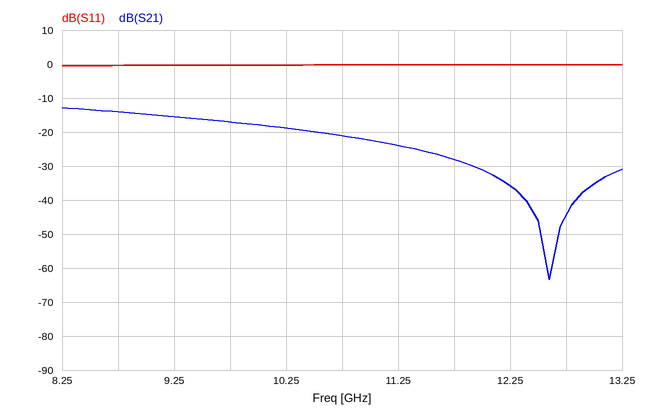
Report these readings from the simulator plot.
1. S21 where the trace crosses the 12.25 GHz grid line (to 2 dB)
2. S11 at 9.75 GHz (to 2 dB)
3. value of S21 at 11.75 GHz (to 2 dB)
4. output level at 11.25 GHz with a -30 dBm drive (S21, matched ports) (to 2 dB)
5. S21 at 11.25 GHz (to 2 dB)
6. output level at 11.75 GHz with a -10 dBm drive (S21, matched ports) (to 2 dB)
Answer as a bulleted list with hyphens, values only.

- -36 dB
- 0 dB
- -28 dB
- -54 dBm
- -24 dB
- -38 dBm
